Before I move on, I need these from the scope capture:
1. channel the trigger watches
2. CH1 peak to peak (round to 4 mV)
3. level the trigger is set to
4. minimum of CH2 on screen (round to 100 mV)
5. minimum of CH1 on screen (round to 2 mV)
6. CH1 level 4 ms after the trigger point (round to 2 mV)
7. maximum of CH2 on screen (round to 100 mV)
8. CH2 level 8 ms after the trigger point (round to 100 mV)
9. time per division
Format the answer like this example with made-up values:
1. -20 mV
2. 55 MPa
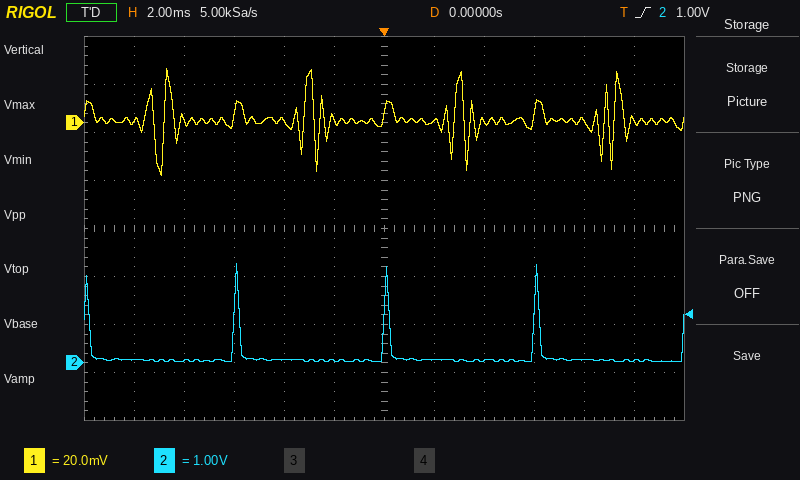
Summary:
1. CH2
2. 44 mV
3. 1.00 V
4. 0.0 V
5. -22 mV
6. 0 mV
7. 2.1 V
8. 100 mV
9. 2 ms
